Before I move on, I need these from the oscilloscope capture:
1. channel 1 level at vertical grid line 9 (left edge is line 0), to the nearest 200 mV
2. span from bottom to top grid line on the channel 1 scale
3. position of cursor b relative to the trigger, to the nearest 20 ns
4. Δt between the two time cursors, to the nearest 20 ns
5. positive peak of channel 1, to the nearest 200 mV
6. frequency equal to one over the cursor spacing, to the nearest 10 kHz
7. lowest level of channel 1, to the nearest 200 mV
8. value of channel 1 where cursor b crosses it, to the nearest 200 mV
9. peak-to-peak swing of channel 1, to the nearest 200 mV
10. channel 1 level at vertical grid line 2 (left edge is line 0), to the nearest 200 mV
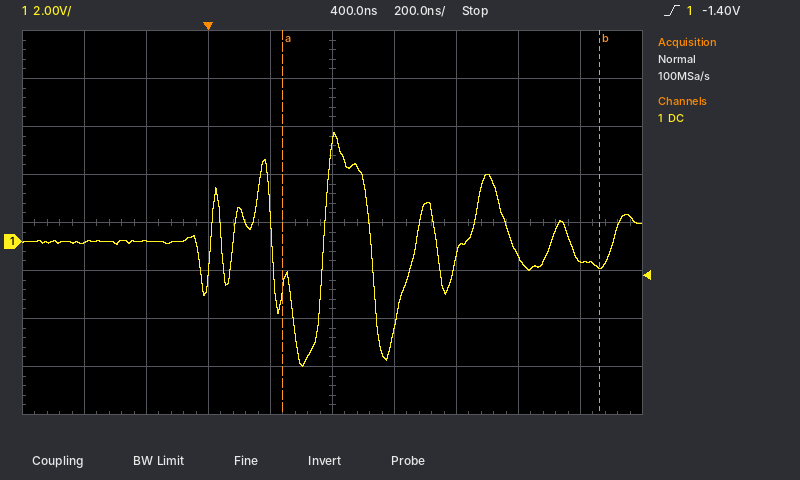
-800 mV
16 V
+1.26 µs
1.02 µs
4.6 V
980 kHz
-5.2 V
-1.0 V
9.8 V
0.0 V
